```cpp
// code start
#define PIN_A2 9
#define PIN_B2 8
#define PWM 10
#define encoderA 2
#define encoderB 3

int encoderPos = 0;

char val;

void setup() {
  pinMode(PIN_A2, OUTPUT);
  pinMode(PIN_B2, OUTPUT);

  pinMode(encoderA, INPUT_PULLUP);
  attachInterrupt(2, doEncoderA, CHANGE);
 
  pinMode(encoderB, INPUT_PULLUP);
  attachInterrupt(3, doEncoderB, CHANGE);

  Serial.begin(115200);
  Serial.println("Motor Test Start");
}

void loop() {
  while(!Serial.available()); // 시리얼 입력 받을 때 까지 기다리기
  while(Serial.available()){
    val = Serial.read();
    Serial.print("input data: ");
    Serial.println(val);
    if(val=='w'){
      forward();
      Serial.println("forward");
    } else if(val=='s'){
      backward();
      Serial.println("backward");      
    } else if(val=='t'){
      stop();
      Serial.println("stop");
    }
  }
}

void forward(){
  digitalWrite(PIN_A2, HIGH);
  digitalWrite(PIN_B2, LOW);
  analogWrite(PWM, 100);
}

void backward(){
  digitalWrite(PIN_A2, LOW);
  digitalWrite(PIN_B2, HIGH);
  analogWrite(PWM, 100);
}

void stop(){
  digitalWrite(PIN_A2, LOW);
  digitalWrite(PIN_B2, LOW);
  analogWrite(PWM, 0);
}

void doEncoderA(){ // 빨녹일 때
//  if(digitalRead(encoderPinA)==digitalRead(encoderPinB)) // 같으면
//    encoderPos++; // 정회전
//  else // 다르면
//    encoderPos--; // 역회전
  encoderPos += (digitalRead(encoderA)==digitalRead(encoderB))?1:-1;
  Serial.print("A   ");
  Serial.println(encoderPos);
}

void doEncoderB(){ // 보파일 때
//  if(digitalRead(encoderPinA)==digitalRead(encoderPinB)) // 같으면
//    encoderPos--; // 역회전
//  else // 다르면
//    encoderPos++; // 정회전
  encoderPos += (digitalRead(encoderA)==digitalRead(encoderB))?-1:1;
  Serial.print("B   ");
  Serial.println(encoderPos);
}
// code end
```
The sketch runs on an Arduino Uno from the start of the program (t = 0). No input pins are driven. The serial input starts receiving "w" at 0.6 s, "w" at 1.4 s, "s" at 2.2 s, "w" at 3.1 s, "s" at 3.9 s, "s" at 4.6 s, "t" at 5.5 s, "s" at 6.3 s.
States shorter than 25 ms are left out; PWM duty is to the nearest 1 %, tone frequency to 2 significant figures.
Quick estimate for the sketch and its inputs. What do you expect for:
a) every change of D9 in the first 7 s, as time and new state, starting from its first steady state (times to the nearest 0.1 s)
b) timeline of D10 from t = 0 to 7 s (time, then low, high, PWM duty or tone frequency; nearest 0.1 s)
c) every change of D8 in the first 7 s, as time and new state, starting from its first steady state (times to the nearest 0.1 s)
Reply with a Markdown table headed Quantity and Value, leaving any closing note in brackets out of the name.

| Quantity | Value |
|---|---|
| every change of D9 in the first 7 s, as time and new state, starting from its first steady state | 0 s low; 0.6 s high; 2.2 s low; 3.1 s high; 3.9 s low |
| timeline of D10 from t = 0 to 7 s | 0.6 s PWM 39 %; 5.5 s low; 6.3 s PWM 39 % |
| every change of D8 in the first 7 s, as time and new state, starting from its first steady state | 0 s low; 2.2 s high; 3.1 s low; 3.9 s high; 5.5 s low; 6.3 s high |
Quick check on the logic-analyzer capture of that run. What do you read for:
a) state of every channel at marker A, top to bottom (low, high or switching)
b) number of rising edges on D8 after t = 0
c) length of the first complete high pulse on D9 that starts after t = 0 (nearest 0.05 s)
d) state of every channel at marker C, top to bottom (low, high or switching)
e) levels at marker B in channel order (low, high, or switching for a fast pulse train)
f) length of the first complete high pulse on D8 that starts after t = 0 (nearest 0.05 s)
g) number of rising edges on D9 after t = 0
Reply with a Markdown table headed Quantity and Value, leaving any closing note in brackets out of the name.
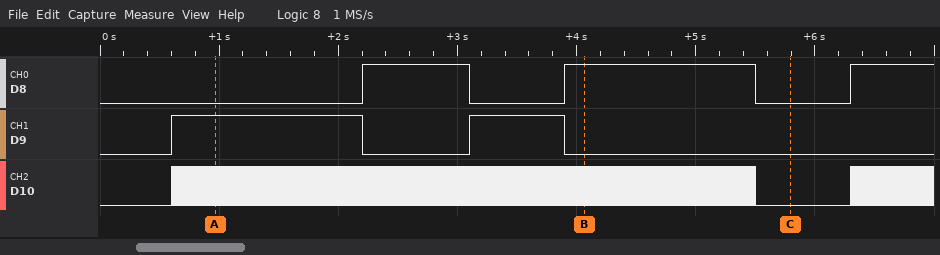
| Quantity | Value |
|---|---|
| state of every channel at marker A, top to bottom | D8 low, D9 high, D10 switching |
| number of rising edges on D8 after t = 0 | 3 |
| length of the first complete high pulse on D9 that starts after t = 0 | 1.60 s |
| state of every channel at marker C, top to bottom | D8 low, D9 low, D10 low |
| levels at marker B in channel order | D8 high, D9 low, D10 switching |
| length of the first complete high pulse on D8 that starts after t = 0 | 0.90 s |
| number of rising edges on D9 after t = 0 | 2 |
